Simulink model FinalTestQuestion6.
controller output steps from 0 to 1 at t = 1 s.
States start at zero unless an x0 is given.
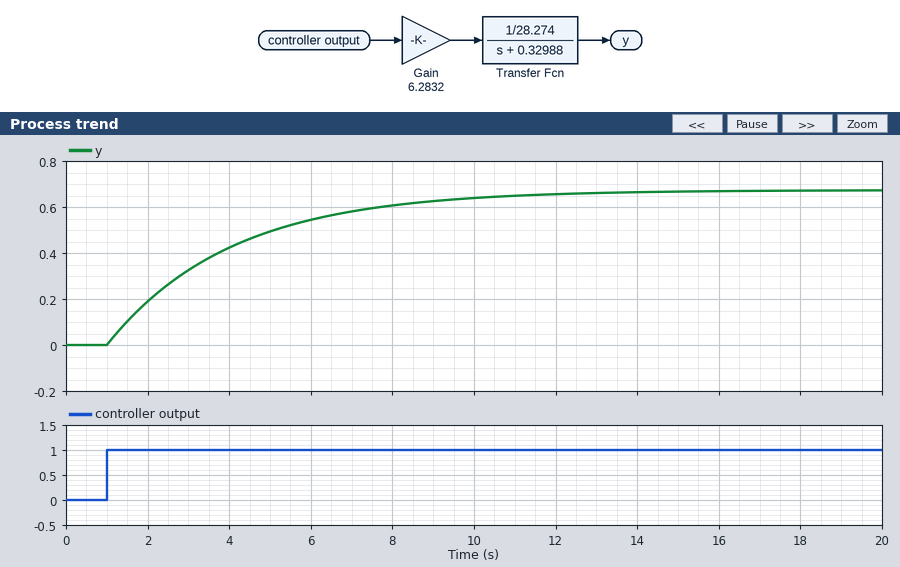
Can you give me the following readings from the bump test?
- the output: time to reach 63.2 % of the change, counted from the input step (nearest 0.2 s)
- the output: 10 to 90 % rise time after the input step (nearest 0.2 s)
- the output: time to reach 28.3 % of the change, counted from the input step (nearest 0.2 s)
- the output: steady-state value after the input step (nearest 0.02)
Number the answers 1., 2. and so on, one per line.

1. 3.0 s
2. 6.6 s
3. 1.0 s
4. 0.68
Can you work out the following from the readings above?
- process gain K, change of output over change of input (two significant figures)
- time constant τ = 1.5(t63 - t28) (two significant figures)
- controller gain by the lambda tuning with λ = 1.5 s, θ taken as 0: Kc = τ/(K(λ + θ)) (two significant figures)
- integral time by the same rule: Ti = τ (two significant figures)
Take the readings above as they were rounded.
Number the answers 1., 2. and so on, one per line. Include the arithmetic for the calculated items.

1. (0.68 - 0) / 1 = 0.68
2. 1.5 × (3 - 1) = 3.0 s
3. 3 / (0.68 × (1.5 + 0)) = 2.9
4. 3.0 s
